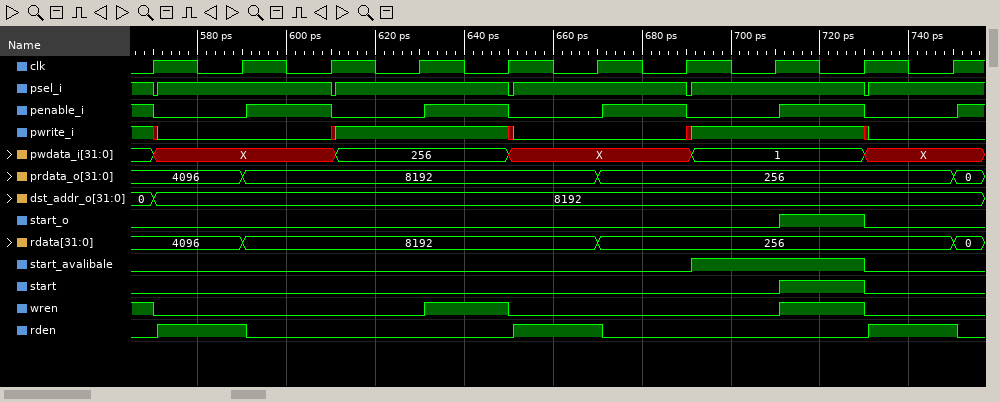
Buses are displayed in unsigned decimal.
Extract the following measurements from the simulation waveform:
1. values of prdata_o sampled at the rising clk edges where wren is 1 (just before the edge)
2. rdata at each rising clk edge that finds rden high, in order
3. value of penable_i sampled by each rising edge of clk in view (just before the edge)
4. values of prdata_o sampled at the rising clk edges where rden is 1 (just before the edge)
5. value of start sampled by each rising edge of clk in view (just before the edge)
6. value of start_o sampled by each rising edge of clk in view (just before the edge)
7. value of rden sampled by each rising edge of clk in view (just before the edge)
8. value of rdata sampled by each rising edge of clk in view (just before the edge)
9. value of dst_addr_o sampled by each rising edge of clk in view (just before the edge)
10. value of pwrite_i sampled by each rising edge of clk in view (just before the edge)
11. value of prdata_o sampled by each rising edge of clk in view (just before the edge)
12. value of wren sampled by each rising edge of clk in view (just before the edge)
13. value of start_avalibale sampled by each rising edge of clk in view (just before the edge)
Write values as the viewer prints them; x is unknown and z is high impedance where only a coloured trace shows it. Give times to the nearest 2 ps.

4096, 8192, 256
4096, 8192, 256
1 0 1 0 1 0 1 0 1 0
4096, 8192, 256
0 0 0 0 0 0 0 0 1 0
0 0 0 0 0 0 0 0 1 0
0 1 0 0 0 1 0 0 0 1
4096, 4096, 8192, 8192, 8192, 8192, 256, 256, 256, 256
0, 8192, 8192, 8192, 8192, 8192, 8192, 8192, 8192, 8192
1 0 0 1 1 0 0 1 1 0
4096, 4096, 8192, 8192, 8192, 8192, 256, 256, 256, 256
1 0 0 0 1 0 0 0 1 0
0 0 0 0 0 0 0 1 1 0
